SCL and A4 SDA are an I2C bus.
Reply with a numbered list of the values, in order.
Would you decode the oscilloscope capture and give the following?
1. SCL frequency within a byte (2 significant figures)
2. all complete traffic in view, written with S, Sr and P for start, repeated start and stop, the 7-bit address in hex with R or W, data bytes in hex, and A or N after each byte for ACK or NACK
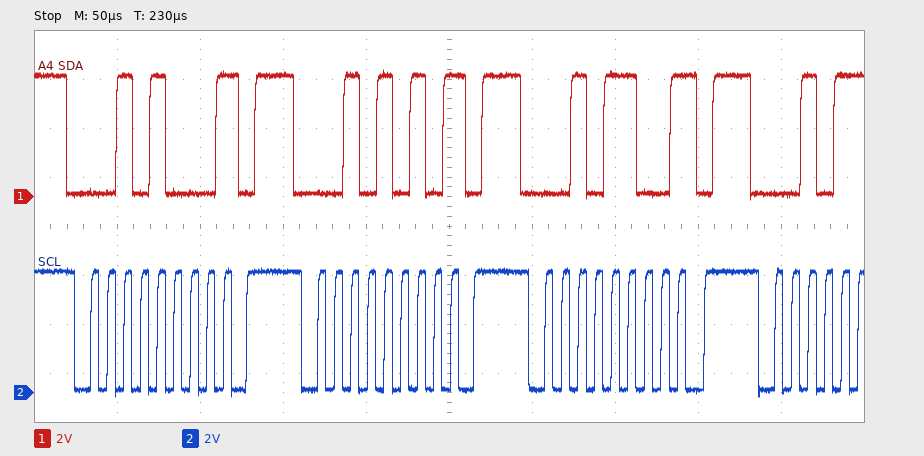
1. 100 kHz
2. S 14W N P S 15W N P S 16W N P
